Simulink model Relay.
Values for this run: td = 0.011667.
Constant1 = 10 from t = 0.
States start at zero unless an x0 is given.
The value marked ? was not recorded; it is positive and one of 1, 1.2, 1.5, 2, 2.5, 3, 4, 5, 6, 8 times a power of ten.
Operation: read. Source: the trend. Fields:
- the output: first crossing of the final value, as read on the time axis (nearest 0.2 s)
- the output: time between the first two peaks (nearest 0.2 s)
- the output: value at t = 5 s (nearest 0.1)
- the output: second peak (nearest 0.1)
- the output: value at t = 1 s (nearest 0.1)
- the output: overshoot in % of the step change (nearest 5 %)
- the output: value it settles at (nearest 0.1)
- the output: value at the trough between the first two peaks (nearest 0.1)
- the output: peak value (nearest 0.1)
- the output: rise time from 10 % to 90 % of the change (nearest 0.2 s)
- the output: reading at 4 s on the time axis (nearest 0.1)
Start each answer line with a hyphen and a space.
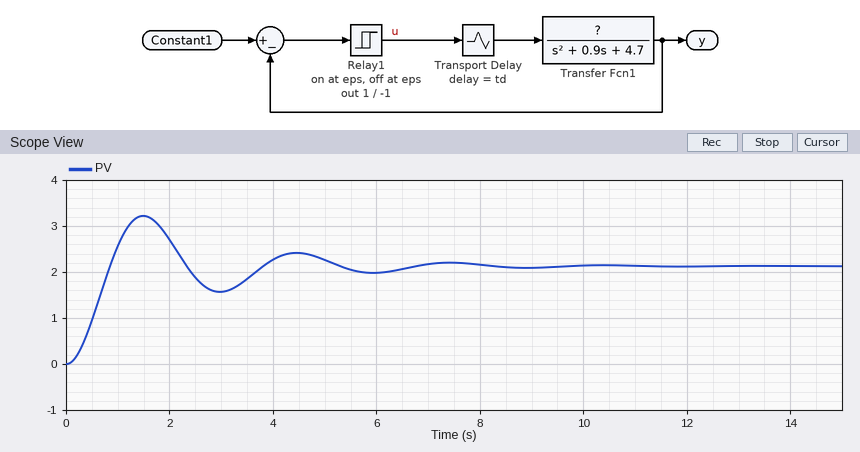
- 0.8 s
- 3.0 s
- 2.3
- 2.4
- 2.6
- 50 %
- 2.1
- 1.6
- 3.2
- 0.6 s
- 2.3
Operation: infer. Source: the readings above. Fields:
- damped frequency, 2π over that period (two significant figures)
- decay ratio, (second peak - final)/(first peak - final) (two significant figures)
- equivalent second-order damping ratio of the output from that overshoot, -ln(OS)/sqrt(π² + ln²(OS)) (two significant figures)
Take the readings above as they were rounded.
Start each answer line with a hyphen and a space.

- 2.1 rad/s
- 0.27
- 0.22
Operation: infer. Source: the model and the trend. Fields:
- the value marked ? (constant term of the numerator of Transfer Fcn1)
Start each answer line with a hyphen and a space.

- 10
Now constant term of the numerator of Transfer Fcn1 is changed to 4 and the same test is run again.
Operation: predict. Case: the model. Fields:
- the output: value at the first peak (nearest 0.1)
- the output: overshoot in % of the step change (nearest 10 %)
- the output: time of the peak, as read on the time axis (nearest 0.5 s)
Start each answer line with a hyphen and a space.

- 1.3
- 50 %
- 1.5 s
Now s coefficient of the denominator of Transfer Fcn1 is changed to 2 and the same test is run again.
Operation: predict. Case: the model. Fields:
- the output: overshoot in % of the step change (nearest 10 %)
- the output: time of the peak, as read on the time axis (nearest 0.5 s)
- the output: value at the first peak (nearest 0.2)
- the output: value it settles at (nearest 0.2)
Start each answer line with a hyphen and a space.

- 20 %
- 1.5 s
- 2.6
- 2.2
